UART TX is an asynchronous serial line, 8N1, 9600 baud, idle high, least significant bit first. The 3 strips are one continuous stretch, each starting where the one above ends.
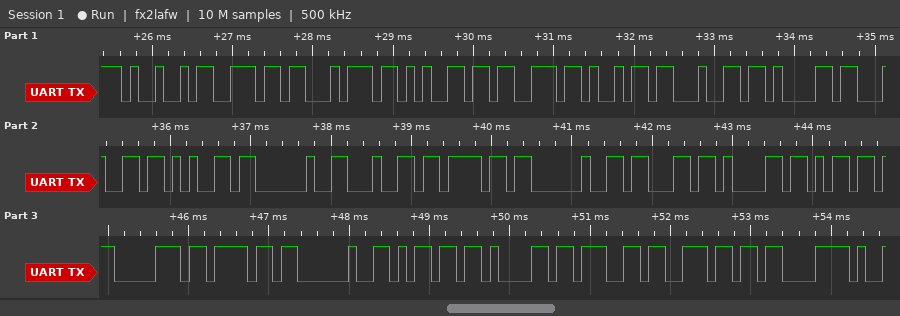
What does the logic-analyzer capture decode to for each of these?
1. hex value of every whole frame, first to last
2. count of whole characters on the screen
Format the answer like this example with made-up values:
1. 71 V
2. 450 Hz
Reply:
1. 0x49 0x6E 0x74 0x65 0x73 0x69 0x64 0x61 0x64 0x65 0x20 0x64 0x6F 0x20 0x63 0x61 0x6D 0x70 0x6F 0x20 0x6D 0x61 0x67 0x6E 0xC3
2. 25
